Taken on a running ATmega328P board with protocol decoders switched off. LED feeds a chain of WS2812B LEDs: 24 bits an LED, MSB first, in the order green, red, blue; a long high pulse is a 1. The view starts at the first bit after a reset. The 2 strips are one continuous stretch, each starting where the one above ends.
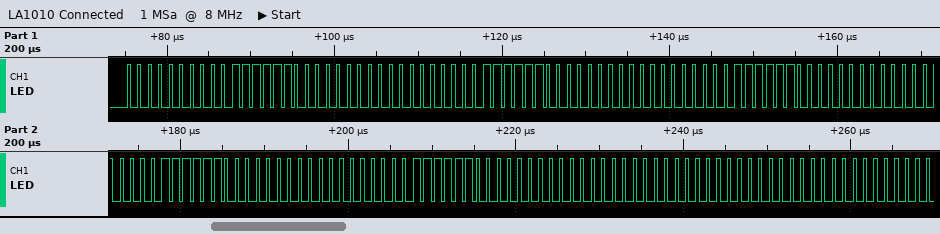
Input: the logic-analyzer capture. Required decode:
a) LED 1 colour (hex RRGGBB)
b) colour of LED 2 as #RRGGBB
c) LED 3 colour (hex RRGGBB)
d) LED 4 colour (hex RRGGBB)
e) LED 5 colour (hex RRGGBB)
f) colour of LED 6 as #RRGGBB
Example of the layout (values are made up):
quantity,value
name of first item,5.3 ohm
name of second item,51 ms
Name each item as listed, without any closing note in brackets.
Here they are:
quantity,value
LED 1 colour,#3F0000
colour of LED 2 as #RRGGBB,#3F0000
LED 3 colour,#3F0000
LED 4 colour,#3F0000
LED 5 colour,#3F0000
colour of LED 6 as #RRGGBB,#000000
